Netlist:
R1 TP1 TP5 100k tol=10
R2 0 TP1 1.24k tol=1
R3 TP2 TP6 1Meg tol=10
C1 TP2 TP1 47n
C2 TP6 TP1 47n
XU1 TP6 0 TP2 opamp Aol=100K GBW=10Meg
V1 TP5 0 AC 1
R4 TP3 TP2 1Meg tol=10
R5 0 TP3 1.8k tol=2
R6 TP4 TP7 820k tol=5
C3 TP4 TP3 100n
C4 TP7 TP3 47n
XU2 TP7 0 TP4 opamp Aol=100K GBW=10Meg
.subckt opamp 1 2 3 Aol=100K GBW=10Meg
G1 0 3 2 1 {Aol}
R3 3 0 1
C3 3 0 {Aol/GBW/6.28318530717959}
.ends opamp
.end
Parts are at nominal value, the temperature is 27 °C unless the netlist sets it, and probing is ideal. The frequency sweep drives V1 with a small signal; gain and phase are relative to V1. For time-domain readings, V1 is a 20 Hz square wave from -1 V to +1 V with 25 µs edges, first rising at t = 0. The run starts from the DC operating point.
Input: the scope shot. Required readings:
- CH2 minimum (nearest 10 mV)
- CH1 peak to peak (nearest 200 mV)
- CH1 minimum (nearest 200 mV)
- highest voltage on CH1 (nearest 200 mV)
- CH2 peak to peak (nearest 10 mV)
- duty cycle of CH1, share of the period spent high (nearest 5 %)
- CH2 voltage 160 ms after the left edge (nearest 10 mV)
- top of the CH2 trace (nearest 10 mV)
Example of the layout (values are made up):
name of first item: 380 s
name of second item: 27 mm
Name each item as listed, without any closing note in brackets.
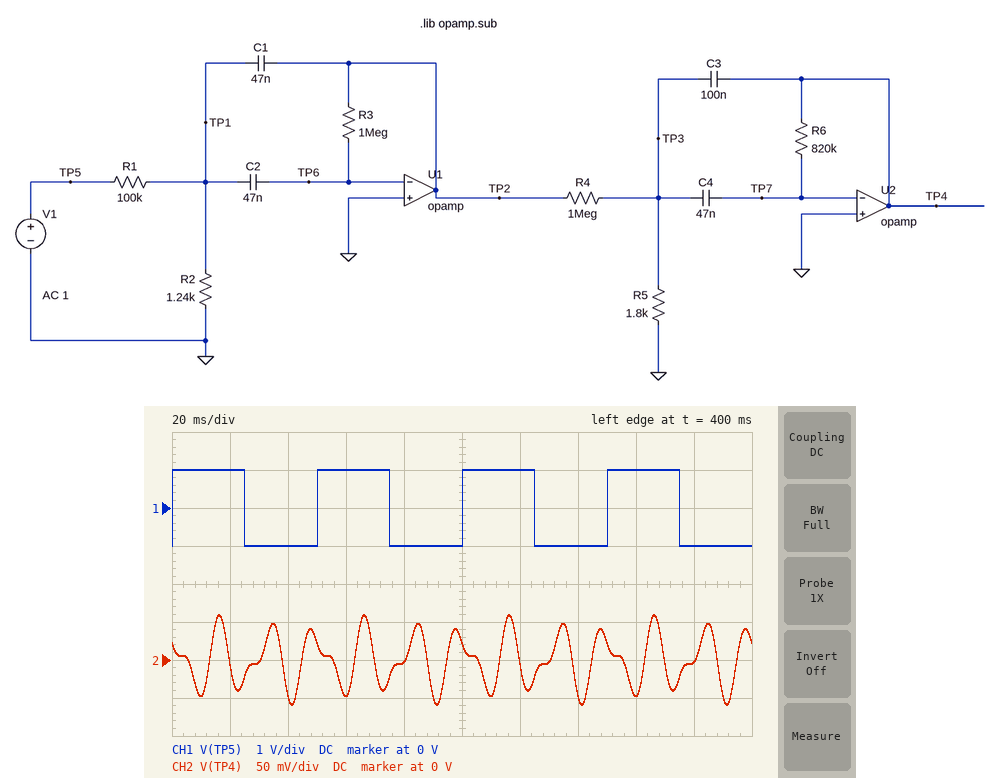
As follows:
CH2 minimum: -60 mV
CH1 peak to peak: 2.0 V
CH1 minimum: -1.0 V
highest voltage on CH1: 1.0 V
CH2 peak to peak: 120 mV
duty cycle of CH1, share of the period spent high: 50 %
CH2 voltage 160 ms after the left edge: -50 mV
top of the CH2 trace: 60 mV
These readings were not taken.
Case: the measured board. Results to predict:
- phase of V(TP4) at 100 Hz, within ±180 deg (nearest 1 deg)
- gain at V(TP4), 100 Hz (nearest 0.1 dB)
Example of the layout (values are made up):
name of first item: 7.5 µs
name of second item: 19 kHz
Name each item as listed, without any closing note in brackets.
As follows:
phase of V(TP4) at 100 Hz, within ±180 deg: -128 deg
gain at V(TP4), 100 Hz: -20.9 dB
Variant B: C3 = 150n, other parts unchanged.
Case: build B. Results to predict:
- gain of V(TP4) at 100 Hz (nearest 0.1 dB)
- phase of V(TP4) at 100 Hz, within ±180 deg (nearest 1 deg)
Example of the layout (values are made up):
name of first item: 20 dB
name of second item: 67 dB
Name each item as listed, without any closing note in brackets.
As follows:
gain of V(TP4) at 100 Hz: -25.9 dB
phase of V(TP4) at 100 Hz, within ±180 deg: -129 deg
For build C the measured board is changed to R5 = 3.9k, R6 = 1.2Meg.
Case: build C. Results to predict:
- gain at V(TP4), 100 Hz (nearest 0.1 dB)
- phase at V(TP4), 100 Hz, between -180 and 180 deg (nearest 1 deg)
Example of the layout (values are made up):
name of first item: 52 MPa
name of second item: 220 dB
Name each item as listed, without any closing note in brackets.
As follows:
gain at V(TP4), 100 Hz: -23.7 dB
phase at V(TP4), 100 Hz, between -180 and 180 deg: -131 deg
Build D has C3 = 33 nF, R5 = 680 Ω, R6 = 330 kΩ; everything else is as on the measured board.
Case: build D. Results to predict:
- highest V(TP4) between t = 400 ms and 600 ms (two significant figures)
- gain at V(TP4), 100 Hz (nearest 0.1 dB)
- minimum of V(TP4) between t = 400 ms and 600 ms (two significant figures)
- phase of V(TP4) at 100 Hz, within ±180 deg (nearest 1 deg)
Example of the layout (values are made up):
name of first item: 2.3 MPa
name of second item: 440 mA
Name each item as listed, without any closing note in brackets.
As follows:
highest V(TP4) between t = 400 ms and 600 ms: 12 mV
gain at V(TP4), 100 Hz: -31.1 dB
minimum of V(TP4) between t = 400 ms and 600 ms: -12 mV
phase of V(TP4) at 100 Hz, within ±180 deg: 44 deg
